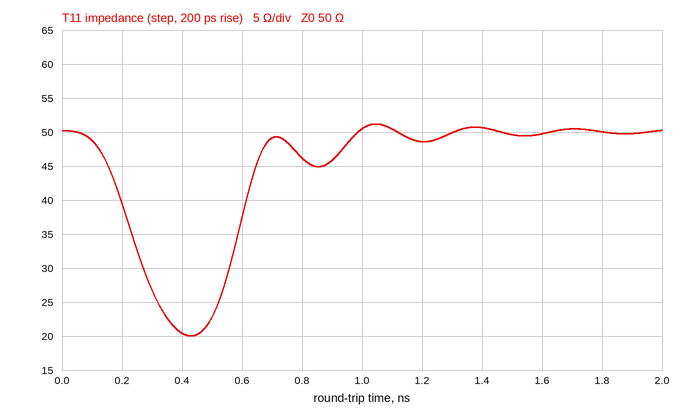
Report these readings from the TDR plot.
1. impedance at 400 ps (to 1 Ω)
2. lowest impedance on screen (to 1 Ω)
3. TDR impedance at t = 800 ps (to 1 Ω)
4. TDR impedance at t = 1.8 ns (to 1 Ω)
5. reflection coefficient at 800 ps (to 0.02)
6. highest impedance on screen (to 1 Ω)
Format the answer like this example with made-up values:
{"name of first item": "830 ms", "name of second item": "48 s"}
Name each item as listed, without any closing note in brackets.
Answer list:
{"impedance at 400 ps": "20 Ω", "lowest impedance on screen": "20 Ω", "TDR impedance at t = 800 ps": "46 Ω", "TDR impedance at t = 1.8 ns": "50 Ω", "reflection coefficient at 800 ps": "-0.04", "highest impedance on screen": "51 Ω"}
